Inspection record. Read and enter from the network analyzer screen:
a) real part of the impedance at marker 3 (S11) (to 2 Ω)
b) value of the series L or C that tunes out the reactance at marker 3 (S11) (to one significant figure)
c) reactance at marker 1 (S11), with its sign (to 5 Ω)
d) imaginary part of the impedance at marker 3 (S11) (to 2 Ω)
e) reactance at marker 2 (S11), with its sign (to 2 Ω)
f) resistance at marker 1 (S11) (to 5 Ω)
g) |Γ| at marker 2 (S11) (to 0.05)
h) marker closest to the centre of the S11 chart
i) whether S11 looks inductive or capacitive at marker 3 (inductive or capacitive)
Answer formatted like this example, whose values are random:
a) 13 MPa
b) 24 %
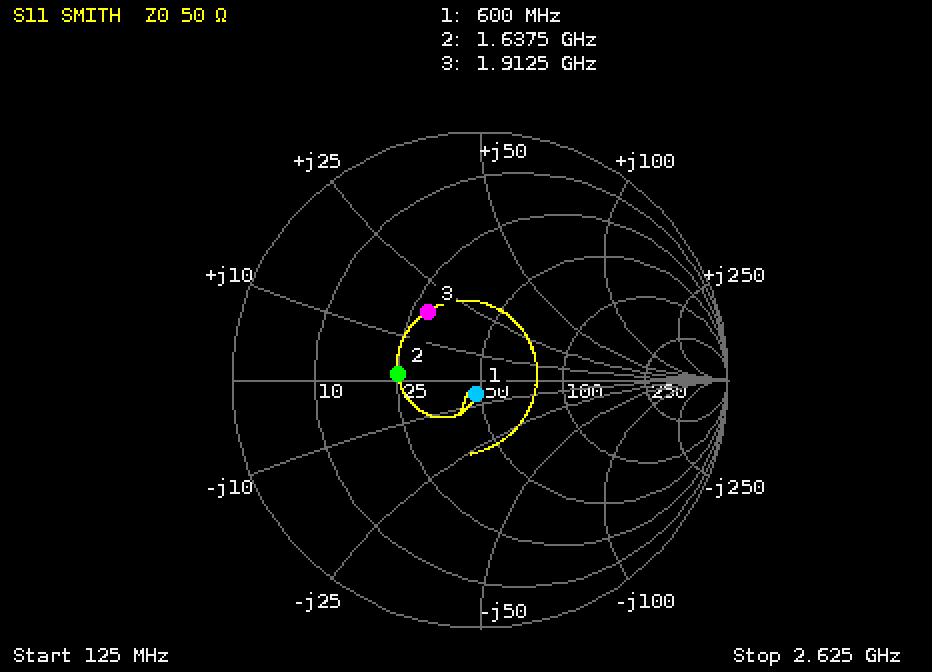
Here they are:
a) 28 Ω
b) 5 pF
c) -5 Ω
d) +18 Ω
e) +2 Ω
f) 50 Ω
g) 0.35
h) marker 1
i) inductive
